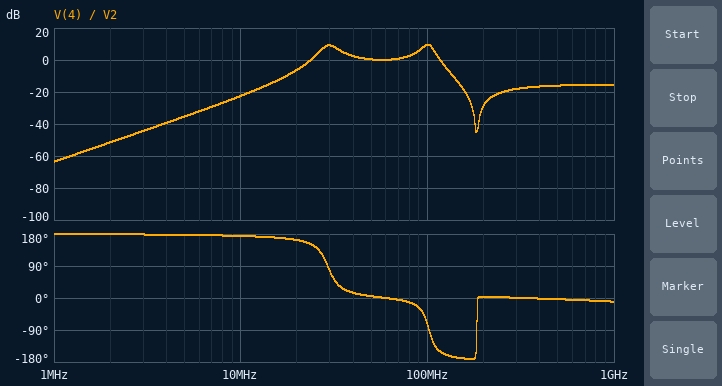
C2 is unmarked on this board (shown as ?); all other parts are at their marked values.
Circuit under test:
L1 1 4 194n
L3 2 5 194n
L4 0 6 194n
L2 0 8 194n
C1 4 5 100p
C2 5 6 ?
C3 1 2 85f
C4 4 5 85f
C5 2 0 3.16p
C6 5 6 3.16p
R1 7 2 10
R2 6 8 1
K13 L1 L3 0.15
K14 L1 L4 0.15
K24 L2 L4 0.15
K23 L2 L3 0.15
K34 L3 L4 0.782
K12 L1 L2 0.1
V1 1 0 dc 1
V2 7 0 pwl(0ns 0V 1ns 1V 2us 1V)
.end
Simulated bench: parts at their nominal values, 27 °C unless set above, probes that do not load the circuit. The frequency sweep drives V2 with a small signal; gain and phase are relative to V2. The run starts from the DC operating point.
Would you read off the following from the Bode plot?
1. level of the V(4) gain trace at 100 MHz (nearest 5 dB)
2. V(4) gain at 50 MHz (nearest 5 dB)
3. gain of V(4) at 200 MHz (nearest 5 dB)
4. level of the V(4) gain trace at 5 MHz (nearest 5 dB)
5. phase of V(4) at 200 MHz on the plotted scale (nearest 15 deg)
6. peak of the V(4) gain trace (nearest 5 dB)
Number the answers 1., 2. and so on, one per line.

1. 10 dB
2. 0 dB
3. -30 dB
4. -35 dB
5. 0 deg
6. 10 dB
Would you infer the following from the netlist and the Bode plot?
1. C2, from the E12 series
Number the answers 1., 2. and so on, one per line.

1. 33 pF
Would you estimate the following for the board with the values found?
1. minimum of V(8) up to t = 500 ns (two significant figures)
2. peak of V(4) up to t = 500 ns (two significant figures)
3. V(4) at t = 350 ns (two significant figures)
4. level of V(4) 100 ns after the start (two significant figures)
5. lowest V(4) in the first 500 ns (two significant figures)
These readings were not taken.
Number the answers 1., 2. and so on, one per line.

1. -450 mV
2. 1.7 V
3. 1.0 V
4. 1.1 V
5. 460 mV
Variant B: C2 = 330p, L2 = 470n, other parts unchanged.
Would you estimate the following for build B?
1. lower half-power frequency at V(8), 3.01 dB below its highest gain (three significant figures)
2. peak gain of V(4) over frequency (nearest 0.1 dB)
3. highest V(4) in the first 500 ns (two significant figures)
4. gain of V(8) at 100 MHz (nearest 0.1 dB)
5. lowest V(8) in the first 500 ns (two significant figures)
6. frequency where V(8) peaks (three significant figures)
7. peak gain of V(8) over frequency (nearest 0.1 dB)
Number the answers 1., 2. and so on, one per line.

1. 33.3 MHz
2. 14.1 dB
3. 1.3 V
4. -11.4 dB
5. -240 mV
6. 34.5 MHz
7. 12.6 dB
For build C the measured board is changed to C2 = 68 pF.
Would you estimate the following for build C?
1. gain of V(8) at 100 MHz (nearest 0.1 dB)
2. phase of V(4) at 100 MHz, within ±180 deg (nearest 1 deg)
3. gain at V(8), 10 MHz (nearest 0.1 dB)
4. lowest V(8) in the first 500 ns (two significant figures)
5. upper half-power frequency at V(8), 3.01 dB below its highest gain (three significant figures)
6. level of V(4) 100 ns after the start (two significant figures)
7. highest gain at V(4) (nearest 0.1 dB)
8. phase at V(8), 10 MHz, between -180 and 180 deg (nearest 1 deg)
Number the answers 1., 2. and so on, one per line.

1. -4.5 dB
2. -160 deg
3. -32.5 dB
4. -380 mV
5. 79.6 MHz
6. 1.1 V
7. 8.6 dB
8. -5 deg
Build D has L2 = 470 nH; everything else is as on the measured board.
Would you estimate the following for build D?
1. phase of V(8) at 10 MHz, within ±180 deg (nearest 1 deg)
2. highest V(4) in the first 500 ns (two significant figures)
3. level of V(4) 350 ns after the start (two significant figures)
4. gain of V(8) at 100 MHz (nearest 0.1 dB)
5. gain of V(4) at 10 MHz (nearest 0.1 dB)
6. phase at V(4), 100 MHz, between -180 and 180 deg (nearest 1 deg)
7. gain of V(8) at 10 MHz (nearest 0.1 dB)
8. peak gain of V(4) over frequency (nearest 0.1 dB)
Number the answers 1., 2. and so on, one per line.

1. -4 deg
2. 1.6 V
3. 1.0 V
4. 10.8 dB
5. -22.6 dB
6. -103 deg
7. -28.4 dB
8. 8.9 dB
